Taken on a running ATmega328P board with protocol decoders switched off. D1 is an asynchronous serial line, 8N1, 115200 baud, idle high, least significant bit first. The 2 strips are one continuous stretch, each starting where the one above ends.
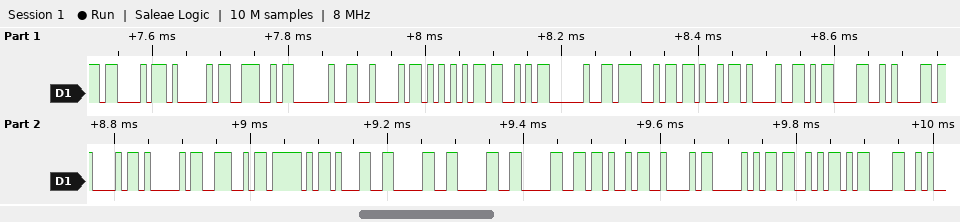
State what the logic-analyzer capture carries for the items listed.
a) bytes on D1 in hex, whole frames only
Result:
43 41 4E 20 42 55 53 20 4F 4B 21 0D 0A 43 41 4E 5F 31 30 30 30 4B 42 50 53 0D
